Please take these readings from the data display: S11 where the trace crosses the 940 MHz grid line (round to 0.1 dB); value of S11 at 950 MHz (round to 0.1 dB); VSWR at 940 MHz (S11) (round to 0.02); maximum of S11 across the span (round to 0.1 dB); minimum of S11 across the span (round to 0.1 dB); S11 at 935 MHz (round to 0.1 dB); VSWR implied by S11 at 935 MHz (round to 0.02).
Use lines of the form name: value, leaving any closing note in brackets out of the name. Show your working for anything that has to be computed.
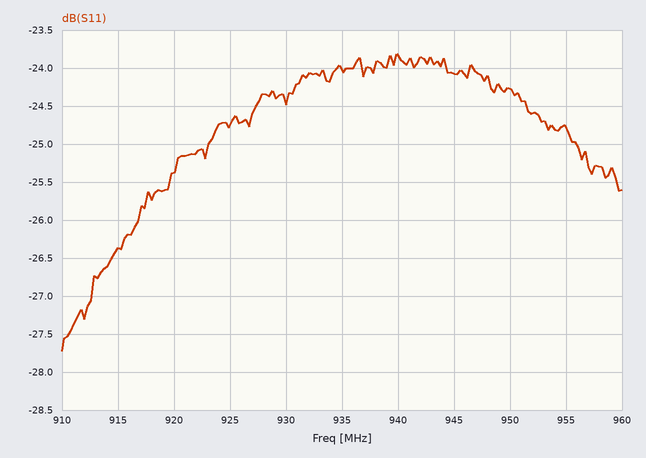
S11 where the trace crosses the 940 MHz grid line: -23.8 dB
value of S11 at 950 MHz: -24.3 dB
VSWR at 940 MHz (S11): |Γ| = 10^(-23.8/20) = 0.0646; VSWR = (1 + 0.0646)/(1 − 0.0646) ≈ 1.14
maximum of S11 across the span: -23.8 dB
minimum of S11 across the span: -27.7 dB
S11 at 935 MHz: -24.0 dB
VSWR implied by S11 at 935 MHz: |Γ| = 10^(-24/20) = 0.0631; VSWR = (1 + 0.0631)/(1 − 0.0631) ≈ 1.13, so 1.14 to the nearest 0.02
